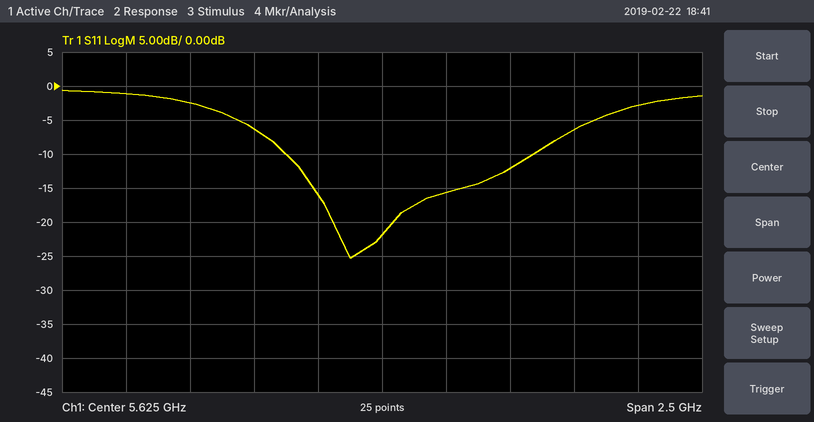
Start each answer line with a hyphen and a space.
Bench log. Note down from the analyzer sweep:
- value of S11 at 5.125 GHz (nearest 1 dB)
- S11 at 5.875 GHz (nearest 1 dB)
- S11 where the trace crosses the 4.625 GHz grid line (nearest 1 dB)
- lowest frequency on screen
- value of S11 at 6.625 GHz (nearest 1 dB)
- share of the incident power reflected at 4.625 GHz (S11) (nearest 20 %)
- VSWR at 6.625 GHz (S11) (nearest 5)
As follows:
- -6 dB
- -16 dB
- -1 dB
- 4.375 GHz
- -3 dB
- 80 %
- 5
